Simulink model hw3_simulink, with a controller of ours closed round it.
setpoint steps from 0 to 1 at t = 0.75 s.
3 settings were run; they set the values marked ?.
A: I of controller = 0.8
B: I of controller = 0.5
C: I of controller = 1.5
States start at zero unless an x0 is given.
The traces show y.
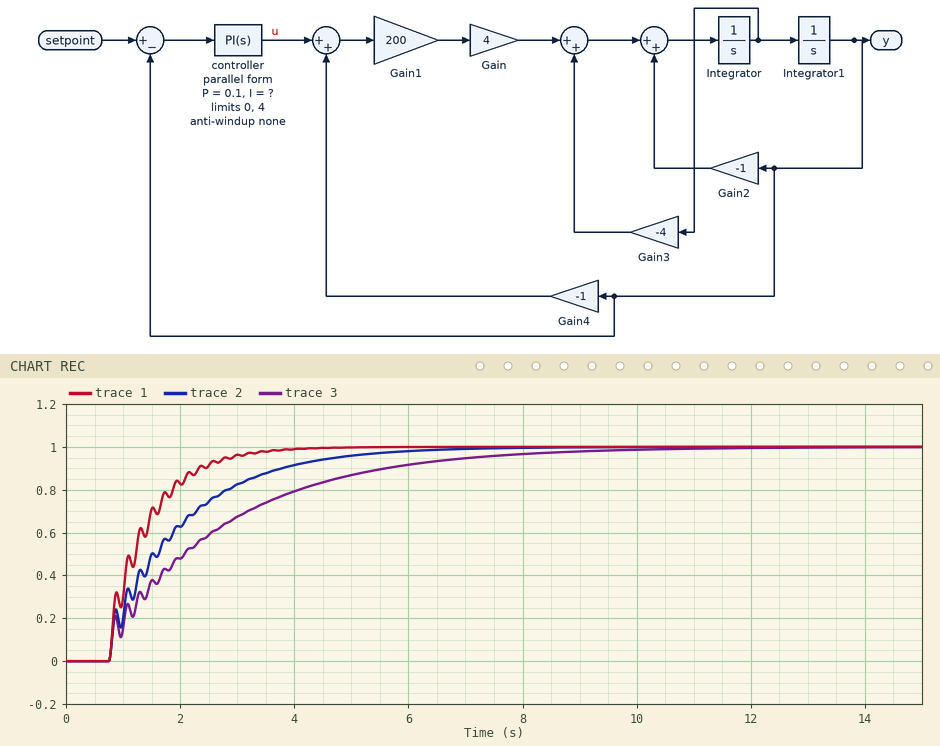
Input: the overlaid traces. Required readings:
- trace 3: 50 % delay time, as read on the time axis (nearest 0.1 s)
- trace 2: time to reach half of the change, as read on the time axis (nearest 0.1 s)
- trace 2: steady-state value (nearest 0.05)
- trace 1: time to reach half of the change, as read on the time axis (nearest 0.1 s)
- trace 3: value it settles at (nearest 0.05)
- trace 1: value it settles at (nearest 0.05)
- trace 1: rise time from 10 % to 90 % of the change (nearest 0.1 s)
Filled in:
2.1 s
1.5 s
1.00
1.2 s
1.00
1.00
1.5 s
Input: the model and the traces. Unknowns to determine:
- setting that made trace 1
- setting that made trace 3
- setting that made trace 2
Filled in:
C
B
A
